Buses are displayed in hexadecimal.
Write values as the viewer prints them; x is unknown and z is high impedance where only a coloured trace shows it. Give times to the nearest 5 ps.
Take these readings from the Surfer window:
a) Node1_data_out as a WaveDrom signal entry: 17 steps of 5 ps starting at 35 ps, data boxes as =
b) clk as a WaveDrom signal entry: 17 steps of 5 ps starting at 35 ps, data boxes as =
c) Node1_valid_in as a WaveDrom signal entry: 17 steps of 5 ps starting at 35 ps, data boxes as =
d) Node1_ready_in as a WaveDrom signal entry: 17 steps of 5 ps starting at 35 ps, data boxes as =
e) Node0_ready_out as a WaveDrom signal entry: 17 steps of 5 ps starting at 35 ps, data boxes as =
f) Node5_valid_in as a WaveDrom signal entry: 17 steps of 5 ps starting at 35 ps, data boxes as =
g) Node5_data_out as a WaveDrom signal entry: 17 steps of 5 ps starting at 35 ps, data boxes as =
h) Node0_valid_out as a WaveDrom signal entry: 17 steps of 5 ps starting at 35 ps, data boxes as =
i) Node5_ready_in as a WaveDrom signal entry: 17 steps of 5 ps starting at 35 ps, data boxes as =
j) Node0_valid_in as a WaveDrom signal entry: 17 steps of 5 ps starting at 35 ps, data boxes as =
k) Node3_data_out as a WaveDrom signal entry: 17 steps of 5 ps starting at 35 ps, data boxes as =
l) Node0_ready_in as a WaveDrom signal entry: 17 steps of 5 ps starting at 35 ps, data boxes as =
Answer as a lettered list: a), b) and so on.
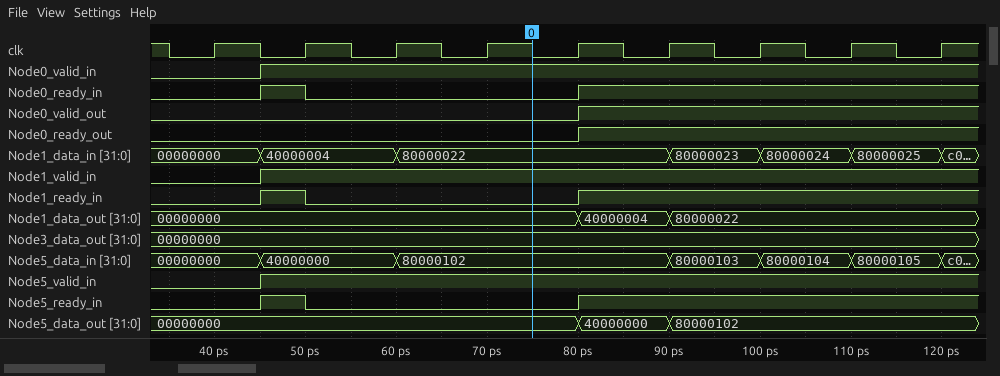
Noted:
a) {name: 'Node1_data_out', wave: '=........=.=.....', data: '00000000 40000004 80000022'}
b) {name: 'clk', wave: '01010101010101010'}
c) {name: 'Node1_valid_in', wave: '0.1..............'}
d) {name: 'Node1_ready_in', wave: '0.10.....1.......'}
e) {name: 'Node0_ready_out', wave: '0........1.......'}
f) {name: 'Node5_valid_in', wave: '0.1..............'}
g) {name: 'Node5_data_out', wave: '=........=.=.....', data: '00000000 40000000 80000102'}
h) {name: 'Node0_valid_out', wave: '0........1.......'}
i) {name: 'Node5_ready_in', wave: '0.10.....1.......'}
j) {name: 'Node0_valid_in', wave: '0.1..............'}
k) {name: 'Node3_data_out', wave: '=................', data: '00000000'}
l) {name: 'Node0_ready_in', wave: '0.10.....1.......'}
